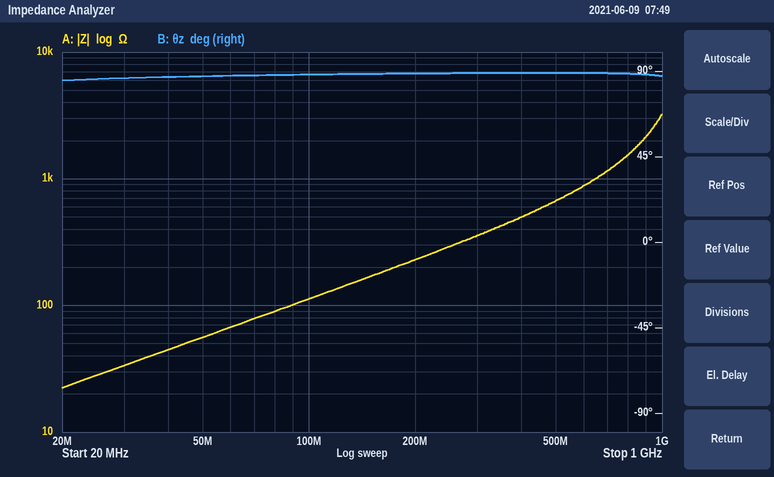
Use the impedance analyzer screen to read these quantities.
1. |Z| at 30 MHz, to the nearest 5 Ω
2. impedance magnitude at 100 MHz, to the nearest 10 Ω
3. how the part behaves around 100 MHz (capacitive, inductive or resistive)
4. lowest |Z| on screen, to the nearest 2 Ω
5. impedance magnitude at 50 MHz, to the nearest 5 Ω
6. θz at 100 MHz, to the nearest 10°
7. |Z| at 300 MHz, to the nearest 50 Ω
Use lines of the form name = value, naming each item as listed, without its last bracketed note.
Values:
|Z| at 30 MHz, to the nearest 5 Ω = 35 Ω
impedance magnitude at 100 MHz, to the nearest 10 Ω = 110 Ω
how the part behaves around 100 MHz = inductive
lowest |Z| on screen, to the nearest 2 Ω = 22 Ω
impedance magnitude at 50 MHz, to the nearest 5 Ω = 55 Ω
θz at 100 MHz, to the nearest 10° = 90°
|Z| at 300 MHz, to the nearest 50 Ω = 350 Ω
